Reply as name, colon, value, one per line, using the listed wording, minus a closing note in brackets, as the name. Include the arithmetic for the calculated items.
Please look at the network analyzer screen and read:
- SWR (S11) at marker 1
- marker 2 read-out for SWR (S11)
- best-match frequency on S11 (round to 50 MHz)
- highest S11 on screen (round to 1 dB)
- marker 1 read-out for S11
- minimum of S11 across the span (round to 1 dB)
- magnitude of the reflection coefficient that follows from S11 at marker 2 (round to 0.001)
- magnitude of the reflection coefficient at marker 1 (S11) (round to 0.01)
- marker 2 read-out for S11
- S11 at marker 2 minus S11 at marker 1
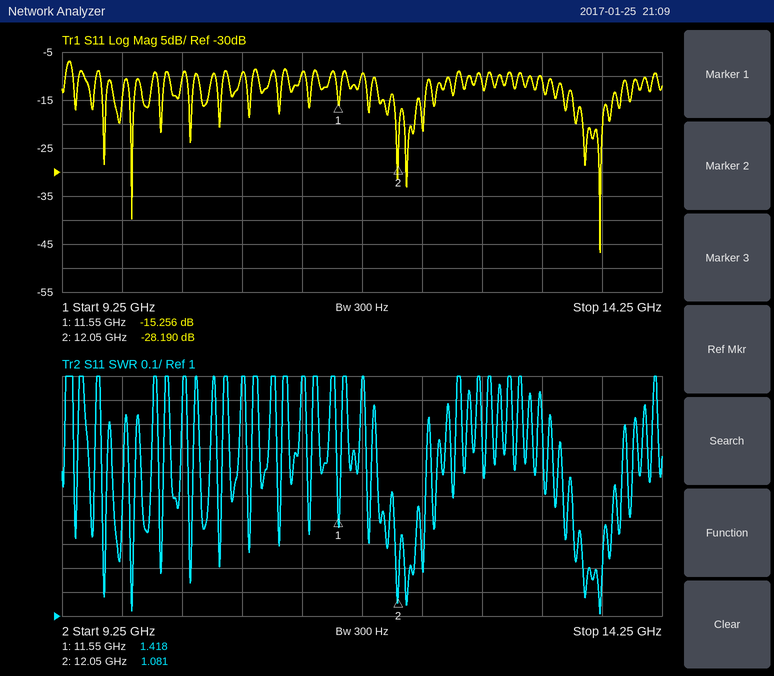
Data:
SWR (S11) at marker 1: 1.418
marker 2 read-out for SWR: 1.081
best-match frequency on S11: 13.75 GHz
highest S11 on screen: -7 dB
marker 1 read-out for S11: -15.256 dB
minimum of S11 across the span: -47 dB
magnitude of the reflection coefficient that follows from S11 at marker 2: 10^(-28.19/20) ≈ 0.039
magnitude of the reflection coefficient at marker 1 (S11): 10^(-15.256/20) ≈ 0.17
marker 2 read-out for S11: -28.190 dB
S11 at marker 2 minus S11 at marker 1: -28.19 − (-15.256) = -12.934 dB
